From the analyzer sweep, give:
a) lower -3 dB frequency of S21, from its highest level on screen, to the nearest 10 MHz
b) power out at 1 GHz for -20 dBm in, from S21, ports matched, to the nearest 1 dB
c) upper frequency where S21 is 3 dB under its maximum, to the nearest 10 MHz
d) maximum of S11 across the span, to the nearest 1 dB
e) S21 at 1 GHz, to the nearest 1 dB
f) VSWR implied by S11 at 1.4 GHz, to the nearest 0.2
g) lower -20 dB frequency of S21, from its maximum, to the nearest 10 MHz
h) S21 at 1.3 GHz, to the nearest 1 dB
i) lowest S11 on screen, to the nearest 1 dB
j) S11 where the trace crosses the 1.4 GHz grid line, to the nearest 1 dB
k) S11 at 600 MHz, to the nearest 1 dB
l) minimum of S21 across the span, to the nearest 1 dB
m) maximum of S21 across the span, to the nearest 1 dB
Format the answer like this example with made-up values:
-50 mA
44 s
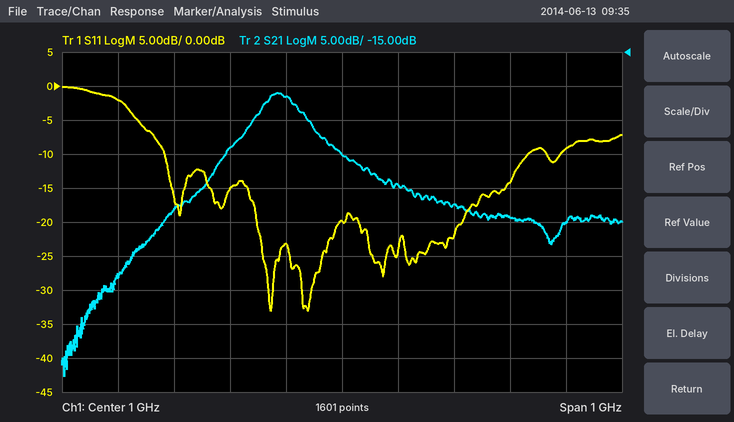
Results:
850 MHz
-50 dBm
930 MHz
0 dB
-30 dB
2.0
670 MHz
-39 dB
-33 dB
-9 dB
-2 dB
-63 dB
-21 dB
